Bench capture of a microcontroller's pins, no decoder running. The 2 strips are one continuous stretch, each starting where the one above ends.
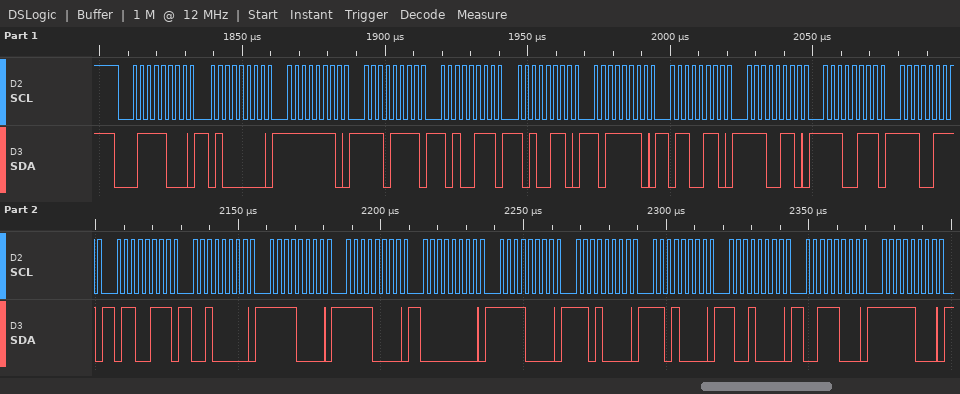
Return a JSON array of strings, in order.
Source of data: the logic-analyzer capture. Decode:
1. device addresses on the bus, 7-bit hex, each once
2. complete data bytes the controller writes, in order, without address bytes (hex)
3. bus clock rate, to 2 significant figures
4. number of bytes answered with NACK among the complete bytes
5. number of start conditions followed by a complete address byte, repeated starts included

["0x3C", "40 FE EF A7 A6 BE 66 E6 E7 E7 67 20 F0 F0 00 F0 D0 D0 90 38 F8", "400 kHz", "0", "1"]
